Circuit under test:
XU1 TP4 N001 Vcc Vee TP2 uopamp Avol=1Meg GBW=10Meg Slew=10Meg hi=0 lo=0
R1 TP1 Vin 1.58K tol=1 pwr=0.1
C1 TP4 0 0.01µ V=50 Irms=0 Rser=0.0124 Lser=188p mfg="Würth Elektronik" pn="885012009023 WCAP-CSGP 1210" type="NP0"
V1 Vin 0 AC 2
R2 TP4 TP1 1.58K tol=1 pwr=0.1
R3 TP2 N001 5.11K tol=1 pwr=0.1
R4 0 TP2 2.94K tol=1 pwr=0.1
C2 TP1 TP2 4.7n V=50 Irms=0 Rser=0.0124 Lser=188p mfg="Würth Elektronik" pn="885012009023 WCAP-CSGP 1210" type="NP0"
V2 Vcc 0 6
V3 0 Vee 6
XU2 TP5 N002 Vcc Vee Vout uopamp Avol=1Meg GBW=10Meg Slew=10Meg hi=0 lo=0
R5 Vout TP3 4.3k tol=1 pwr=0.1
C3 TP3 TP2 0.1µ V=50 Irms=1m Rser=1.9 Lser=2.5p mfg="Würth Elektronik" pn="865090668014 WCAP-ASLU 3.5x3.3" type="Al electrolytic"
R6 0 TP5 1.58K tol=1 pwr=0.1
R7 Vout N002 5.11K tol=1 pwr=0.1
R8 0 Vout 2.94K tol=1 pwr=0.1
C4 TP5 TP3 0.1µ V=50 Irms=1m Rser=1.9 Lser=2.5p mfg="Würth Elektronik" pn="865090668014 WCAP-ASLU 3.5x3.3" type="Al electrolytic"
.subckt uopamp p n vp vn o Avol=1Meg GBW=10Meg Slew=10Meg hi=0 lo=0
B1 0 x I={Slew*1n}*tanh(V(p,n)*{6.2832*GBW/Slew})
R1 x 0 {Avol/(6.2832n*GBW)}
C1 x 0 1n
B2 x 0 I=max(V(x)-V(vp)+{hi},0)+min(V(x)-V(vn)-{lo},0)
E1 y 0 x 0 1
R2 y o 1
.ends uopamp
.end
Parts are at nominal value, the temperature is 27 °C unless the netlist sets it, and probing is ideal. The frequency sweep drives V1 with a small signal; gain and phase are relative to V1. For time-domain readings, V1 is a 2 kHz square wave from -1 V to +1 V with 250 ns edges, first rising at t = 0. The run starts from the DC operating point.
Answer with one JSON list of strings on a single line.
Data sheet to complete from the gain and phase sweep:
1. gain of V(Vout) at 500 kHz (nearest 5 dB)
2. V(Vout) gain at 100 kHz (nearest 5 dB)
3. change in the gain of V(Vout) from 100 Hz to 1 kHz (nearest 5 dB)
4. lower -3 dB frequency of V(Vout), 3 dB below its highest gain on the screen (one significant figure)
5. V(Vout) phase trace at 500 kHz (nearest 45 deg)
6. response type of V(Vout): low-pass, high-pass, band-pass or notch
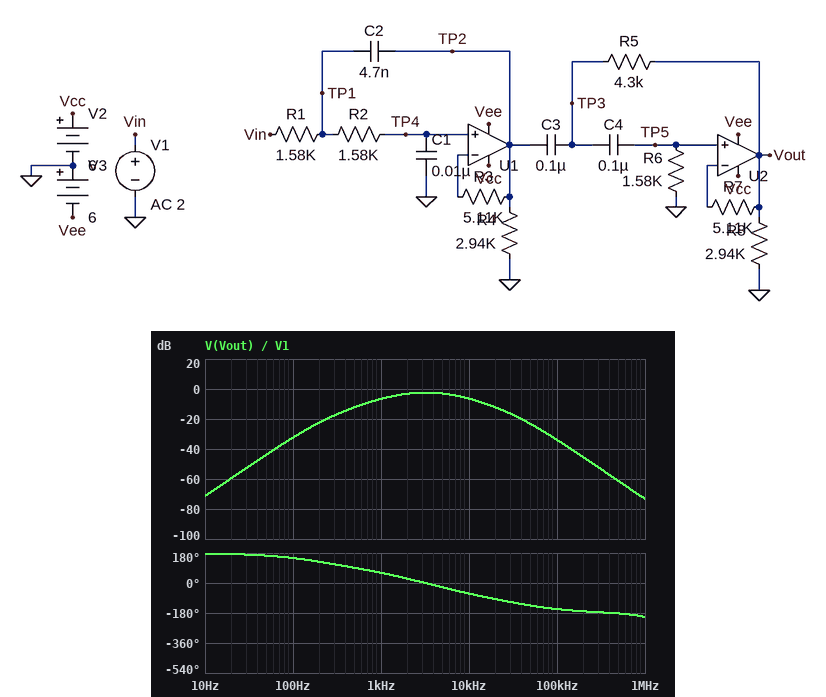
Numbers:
["-60 dB", "-35 dB", "25 dB", "1 kHz", "-180 deg", "band-pass"]
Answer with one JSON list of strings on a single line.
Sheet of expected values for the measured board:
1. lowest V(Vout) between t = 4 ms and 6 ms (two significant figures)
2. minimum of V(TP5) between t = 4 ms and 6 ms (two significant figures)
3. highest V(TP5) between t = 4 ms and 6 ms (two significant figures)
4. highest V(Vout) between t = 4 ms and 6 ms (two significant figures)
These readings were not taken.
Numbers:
["-1.1 V", "-1.1 V", "1.1 V", "1.1 V"]
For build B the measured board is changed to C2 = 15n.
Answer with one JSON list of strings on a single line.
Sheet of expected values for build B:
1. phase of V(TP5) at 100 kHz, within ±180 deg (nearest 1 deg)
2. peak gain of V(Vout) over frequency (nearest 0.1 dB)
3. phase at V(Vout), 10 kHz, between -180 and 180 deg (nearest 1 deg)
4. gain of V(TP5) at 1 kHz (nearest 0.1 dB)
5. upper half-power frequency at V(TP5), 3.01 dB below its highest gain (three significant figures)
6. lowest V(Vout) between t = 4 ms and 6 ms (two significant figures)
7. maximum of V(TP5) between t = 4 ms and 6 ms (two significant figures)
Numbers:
["-172 deg", "-1.7 dB", "-92 deg", "-6.5 dB", "8.41 kHz", "-1.2 V", "1.2 V"]
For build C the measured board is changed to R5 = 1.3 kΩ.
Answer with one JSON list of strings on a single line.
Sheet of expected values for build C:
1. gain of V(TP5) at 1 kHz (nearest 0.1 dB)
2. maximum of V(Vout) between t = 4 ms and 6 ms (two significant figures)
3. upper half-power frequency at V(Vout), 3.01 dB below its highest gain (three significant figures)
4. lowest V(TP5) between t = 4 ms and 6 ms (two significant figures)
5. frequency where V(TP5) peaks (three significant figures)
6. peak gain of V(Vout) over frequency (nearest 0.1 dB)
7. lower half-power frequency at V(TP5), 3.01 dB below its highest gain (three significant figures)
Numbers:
["-6.3 dB", "1.3 V", "7.89 kHz", "-1.3 V", "2.85 kHz", "-1.8 dB", "1.18 kHz"]
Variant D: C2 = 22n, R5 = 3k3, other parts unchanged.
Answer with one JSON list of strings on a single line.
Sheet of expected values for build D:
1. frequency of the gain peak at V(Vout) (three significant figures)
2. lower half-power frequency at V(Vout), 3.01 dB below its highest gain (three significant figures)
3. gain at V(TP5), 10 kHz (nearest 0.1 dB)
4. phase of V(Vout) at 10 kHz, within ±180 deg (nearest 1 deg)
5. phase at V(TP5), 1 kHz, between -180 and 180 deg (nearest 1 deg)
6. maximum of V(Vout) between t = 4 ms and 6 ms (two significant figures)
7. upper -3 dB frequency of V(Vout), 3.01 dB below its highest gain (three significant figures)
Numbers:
["3.98 kHz", "1.44 kHz", "-7.4 dB", "-109 deg", "64 deg", "1.3 V", "7.67 kHz"]
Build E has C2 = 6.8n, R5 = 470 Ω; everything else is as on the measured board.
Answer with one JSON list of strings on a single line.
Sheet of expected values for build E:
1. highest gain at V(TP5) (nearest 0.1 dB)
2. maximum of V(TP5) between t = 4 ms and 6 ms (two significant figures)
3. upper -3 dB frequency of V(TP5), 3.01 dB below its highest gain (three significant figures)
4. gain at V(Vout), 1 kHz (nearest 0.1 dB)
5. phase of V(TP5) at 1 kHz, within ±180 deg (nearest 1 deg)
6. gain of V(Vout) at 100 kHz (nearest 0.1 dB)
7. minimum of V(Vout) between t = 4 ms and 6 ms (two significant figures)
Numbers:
["0 dB", "1.6 V", "6.36 kHz", "-10.1 dB", "129 deg", "-36.8 dB", "-1.6 V"]
